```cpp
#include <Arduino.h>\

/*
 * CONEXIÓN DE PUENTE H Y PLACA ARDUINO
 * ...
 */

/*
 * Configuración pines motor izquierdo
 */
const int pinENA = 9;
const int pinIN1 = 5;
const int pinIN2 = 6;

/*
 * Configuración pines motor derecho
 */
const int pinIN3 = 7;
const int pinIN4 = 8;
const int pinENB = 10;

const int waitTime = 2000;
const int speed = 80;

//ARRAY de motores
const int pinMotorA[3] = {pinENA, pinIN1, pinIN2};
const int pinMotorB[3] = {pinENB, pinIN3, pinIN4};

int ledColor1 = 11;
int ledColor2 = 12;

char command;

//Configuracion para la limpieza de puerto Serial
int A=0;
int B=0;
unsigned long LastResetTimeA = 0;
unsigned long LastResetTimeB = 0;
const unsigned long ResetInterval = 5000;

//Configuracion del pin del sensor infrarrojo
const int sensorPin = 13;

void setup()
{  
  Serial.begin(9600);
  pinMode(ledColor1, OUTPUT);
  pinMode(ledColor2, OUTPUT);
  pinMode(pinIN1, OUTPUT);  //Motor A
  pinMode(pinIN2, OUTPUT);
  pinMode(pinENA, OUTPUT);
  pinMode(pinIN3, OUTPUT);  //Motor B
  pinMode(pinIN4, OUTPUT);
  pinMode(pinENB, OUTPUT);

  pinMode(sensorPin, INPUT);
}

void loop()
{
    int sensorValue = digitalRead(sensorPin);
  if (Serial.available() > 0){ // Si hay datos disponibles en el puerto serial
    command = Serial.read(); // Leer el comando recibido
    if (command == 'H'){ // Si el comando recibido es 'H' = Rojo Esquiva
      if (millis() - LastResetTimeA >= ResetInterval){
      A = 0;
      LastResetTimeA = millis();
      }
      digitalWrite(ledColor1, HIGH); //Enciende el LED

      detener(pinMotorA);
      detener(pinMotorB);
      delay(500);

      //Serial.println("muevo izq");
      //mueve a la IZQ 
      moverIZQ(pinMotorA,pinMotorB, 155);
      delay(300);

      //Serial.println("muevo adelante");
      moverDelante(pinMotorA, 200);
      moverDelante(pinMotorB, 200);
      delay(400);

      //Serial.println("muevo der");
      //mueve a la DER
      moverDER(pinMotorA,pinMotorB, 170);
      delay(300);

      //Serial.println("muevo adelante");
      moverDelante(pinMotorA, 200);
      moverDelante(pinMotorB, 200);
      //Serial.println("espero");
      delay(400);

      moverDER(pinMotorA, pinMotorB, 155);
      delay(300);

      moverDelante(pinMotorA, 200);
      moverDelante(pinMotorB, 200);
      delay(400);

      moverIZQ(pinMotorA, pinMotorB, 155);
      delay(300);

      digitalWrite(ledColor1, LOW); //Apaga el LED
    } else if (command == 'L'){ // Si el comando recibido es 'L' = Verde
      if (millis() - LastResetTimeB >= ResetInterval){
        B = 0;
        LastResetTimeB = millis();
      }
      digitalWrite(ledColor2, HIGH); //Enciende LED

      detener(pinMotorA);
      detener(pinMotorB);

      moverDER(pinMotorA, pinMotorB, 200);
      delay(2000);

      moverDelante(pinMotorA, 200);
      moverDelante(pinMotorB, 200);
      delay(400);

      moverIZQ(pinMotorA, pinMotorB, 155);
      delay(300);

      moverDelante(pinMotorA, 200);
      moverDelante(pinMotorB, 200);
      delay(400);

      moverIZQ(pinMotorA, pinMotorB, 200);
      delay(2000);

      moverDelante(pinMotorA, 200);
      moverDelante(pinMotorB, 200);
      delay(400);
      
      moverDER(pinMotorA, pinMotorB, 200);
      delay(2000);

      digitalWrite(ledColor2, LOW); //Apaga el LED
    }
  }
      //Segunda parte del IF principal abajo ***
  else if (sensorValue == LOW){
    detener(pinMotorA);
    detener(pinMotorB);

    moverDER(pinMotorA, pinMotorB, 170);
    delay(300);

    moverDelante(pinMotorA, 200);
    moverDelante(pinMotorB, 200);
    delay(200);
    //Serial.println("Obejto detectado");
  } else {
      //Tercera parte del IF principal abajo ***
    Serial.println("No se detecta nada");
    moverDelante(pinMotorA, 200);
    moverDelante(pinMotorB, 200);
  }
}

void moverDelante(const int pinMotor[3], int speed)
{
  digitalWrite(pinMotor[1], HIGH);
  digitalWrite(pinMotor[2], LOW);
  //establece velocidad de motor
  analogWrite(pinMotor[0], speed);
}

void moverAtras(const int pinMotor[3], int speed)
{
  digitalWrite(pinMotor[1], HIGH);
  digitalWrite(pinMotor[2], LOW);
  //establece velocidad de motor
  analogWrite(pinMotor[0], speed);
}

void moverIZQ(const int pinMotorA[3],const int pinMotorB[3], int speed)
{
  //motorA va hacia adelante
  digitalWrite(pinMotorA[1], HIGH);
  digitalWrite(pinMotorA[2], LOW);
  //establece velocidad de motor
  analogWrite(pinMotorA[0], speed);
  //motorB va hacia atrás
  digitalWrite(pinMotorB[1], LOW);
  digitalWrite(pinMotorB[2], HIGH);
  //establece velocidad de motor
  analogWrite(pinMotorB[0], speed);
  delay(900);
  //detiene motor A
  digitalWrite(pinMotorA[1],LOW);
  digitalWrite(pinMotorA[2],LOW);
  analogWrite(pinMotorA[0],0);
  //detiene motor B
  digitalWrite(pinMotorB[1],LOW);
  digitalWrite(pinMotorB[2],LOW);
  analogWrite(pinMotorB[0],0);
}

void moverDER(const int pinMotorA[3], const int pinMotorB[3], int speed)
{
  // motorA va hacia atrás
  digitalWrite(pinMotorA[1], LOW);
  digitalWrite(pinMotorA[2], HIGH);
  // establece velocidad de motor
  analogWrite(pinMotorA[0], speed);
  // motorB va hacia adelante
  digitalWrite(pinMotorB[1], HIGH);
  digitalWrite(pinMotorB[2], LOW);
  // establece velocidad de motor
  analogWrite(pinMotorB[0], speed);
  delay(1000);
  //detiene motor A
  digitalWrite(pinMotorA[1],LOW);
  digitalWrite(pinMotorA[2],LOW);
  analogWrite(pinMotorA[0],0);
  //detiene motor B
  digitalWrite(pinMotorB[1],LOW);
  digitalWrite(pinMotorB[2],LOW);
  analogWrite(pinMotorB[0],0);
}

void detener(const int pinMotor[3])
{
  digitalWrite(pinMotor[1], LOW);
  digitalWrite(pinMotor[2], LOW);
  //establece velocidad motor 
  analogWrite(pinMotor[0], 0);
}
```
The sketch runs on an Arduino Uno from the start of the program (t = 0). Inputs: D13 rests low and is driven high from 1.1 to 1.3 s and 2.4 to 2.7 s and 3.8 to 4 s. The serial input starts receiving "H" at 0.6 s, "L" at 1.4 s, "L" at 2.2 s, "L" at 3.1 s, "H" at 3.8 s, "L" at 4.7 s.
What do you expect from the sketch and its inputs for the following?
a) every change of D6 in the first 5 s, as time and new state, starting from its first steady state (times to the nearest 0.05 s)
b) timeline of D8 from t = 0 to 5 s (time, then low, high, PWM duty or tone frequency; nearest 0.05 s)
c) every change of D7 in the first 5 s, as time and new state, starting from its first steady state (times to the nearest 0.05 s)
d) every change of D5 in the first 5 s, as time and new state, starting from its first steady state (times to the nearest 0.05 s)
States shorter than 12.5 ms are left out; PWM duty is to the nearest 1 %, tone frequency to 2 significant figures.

0 s high; 1 s low; 3.6 s high; 4.6 s low
0 s low; 2 s high; 2.9 s low
0 s high; 1 s low; 1.3 s high; 1.5 s low; 3.2 s high; 4.6 s low; 4.9 s high
0 s low; 1.3 s high; 1.5 s low; 2 s high; 2.9 s low; 3.2 s high; 3.6 s low; 4.9 s high
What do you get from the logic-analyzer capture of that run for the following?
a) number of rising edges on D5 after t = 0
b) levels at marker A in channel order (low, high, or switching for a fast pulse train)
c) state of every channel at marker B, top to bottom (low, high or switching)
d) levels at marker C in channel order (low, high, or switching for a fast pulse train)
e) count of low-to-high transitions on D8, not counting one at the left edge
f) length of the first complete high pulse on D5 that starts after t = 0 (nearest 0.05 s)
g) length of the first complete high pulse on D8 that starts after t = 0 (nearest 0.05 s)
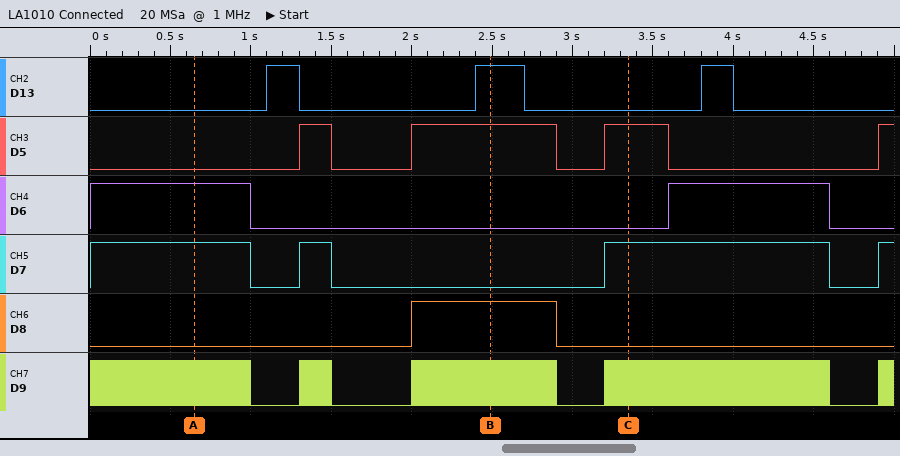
4
D13 low, D5 low, D6 high, D7 high, D8 low, D9 switching
D13 high, D5 high, D6 low, D7 low, D8 high, D9 switching
D13 low, D5 high, D6 low, D7 high, D8 low, D9 switching
1
0.20 s
0.90 s
